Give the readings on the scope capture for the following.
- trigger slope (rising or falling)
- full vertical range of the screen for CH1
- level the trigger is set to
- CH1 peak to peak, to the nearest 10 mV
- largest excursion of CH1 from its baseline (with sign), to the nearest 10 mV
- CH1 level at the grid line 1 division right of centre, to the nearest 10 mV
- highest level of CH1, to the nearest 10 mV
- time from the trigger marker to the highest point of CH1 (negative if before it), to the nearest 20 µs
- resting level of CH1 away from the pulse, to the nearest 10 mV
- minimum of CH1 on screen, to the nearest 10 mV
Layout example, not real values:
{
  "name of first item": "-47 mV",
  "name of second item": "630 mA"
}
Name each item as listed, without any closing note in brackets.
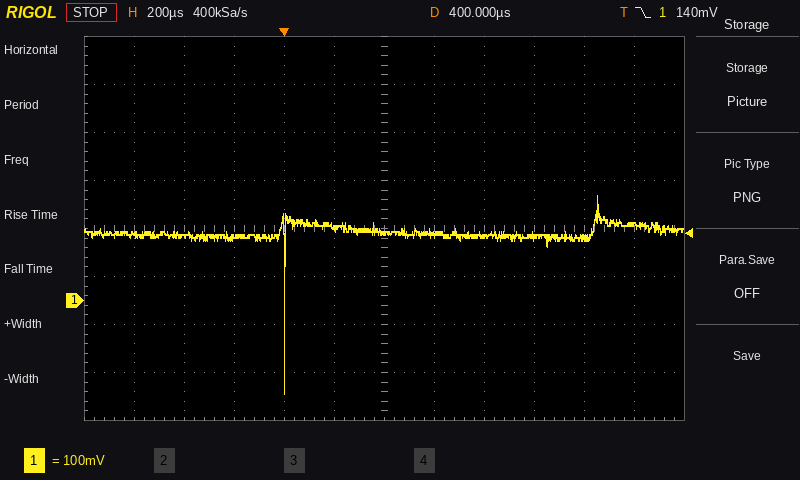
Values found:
{
  "trigger slope": "falling",
  "full vertical range of the screen for CH1": "800 mV",
  "level the trigger is set to": "140 mV",
  "CH1 peak to peak, to the nearest 10 mV": "410 mV",
  "largest excursion of CH1 from its baseline (with sign), to the nearest 10 mV": "-330 mV",
  "CH1 level at the grid line 1 division right of centre, to the nearest 10 mV": "140 mV",
  "highest level of CH1, to the nearest 10 mV": "220 mV",
  "time from the trigger marker to the highest point of CH1 (negative if before it), to the nearest 20 µs": "+1.26 ms",
  "resting level of CH1 away from the pulse, to the nearest 10 mV": "140 mV",
  "minimum of CH1 on screen, to the nearest 10 mV": "-190 mV"
}
